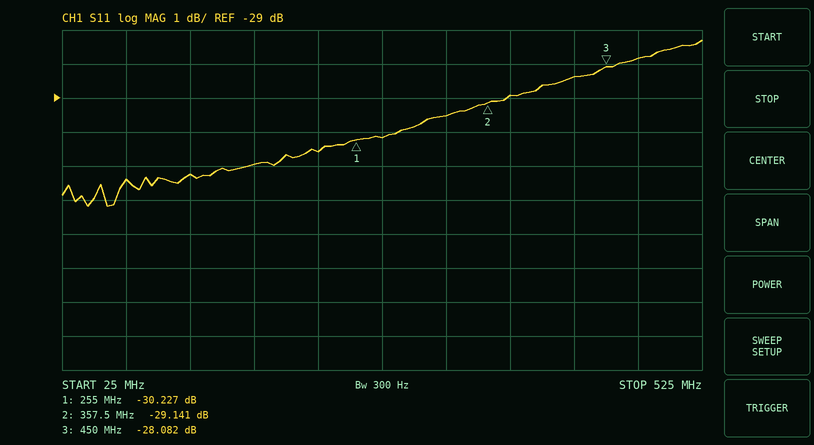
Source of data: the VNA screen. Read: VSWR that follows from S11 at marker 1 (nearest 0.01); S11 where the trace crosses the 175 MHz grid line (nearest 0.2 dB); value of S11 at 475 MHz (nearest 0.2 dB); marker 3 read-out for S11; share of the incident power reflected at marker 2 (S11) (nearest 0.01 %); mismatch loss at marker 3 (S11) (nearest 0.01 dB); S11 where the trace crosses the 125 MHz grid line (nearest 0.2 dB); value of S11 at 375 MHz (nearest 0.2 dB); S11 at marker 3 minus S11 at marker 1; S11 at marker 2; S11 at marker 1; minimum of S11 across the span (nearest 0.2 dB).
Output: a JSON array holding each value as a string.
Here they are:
["1.06", "-31.0 dB", "-27.8 dB", "-28.082 dB", "0.12 %", "0.01 dB", "-31.2 dB", "-29.0 dB", "2.145 dB", "-29.141 dB", "-30.227 dB", "-32.2 dB"]
